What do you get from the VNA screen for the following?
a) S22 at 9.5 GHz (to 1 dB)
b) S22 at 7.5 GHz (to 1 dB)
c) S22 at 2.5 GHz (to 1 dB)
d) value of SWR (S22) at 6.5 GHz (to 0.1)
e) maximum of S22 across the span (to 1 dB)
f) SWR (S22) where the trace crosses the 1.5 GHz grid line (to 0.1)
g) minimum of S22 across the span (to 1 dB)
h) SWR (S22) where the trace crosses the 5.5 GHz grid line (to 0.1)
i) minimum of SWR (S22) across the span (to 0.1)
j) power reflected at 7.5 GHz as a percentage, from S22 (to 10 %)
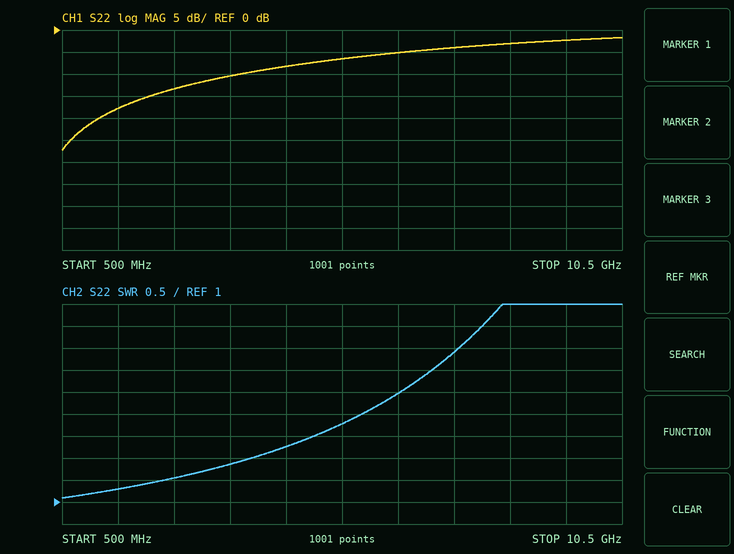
-2 dB
-4 dB
-13 dB
3.5
-2 dB
1.3
-27 dB
2.8
1.1
40 %
